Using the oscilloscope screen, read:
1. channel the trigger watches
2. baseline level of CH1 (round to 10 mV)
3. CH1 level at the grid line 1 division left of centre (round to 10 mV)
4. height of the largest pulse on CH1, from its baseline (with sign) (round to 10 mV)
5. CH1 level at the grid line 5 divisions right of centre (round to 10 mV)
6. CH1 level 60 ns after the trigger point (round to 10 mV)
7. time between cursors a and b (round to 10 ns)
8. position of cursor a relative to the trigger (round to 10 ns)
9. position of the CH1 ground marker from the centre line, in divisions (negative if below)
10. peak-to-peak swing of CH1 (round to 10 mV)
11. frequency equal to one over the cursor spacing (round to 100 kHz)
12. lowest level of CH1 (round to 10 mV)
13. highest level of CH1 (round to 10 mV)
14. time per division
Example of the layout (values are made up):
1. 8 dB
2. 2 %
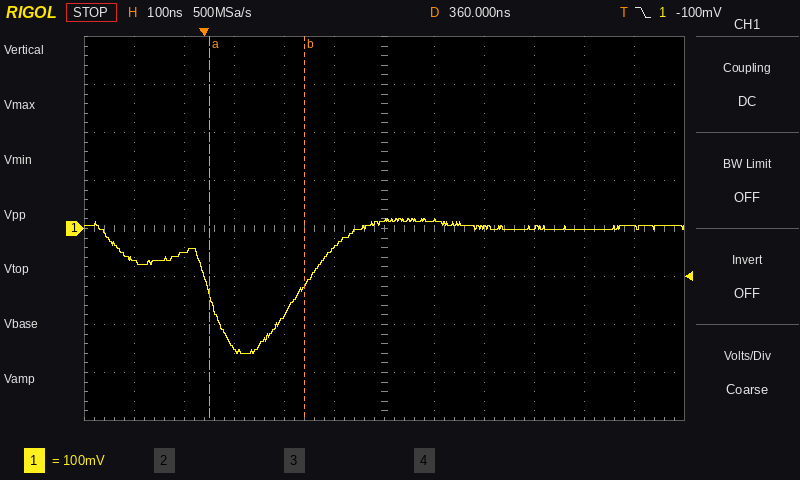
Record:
1. CH1
2. 0 mV
3. -40 mV
4. -260 mV
5. 0 mV
6. -250 mV
7. 190 ns
8. +10 ns
9. 0.0 div
10. 280 mV
11. 5.3 MHz
12. -260 mV
13. 20 mV
14. 100 ns
